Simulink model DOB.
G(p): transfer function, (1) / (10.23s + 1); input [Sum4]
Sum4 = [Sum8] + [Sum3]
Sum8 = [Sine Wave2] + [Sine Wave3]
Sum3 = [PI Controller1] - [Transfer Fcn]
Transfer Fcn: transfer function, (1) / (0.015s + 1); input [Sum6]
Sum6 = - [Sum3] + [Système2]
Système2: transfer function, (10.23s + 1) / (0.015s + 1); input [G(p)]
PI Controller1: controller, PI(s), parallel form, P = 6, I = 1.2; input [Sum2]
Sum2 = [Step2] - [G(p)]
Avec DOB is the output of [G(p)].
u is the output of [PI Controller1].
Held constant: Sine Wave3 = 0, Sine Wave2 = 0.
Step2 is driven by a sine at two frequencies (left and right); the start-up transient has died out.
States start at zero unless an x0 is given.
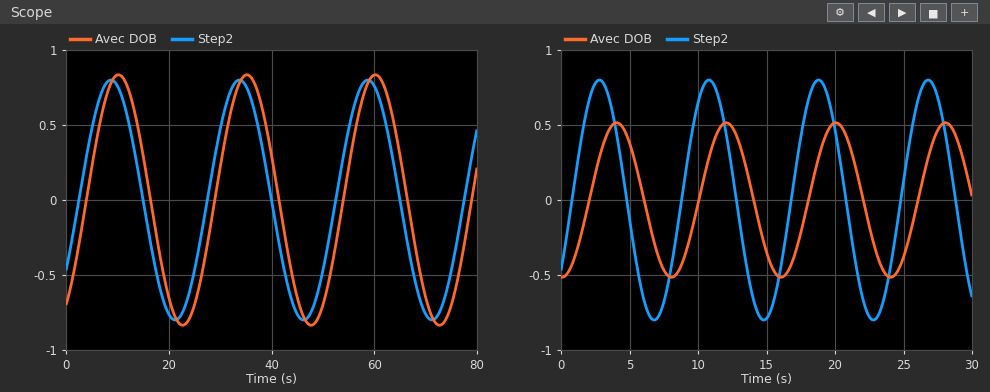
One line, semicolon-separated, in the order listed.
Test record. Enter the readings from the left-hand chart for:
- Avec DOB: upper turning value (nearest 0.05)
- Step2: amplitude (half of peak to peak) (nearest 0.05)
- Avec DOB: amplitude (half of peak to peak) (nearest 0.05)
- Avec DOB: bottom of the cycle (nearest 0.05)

0.85; 0.80; 0.85; -0.85
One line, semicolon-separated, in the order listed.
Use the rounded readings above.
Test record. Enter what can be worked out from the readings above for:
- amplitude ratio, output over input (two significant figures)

1.1
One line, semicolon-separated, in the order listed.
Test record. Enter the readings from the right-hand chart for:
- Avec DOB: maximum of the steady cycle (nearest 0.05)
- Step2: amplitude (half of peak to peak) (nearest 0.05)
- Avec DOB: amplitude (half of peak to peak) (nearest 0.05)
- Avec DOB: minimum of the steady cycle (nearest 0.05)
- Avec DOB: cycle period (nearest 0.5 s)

0.50; 0.80; 0.50; -0.50; 8.0 s
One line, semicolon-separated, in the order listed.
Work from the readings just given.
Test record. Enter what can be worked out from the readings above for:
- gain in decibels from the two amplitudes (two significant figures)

-4.1 dB
